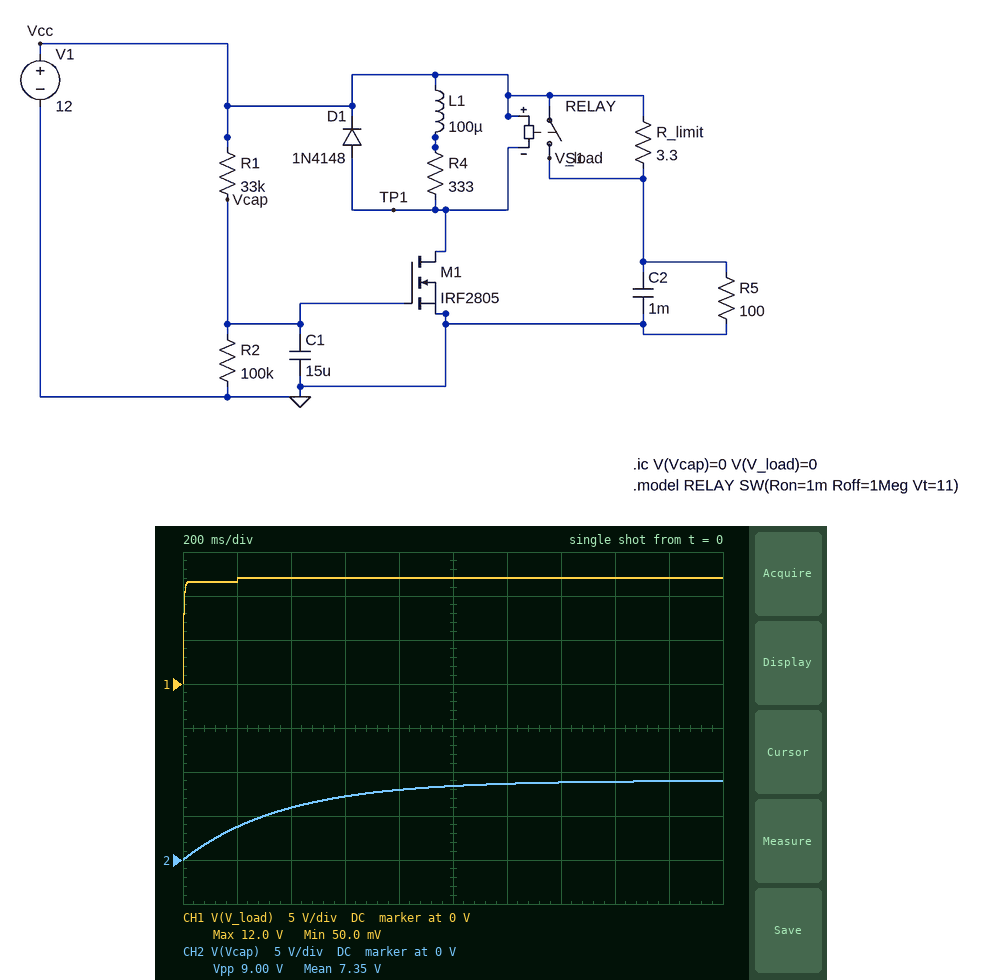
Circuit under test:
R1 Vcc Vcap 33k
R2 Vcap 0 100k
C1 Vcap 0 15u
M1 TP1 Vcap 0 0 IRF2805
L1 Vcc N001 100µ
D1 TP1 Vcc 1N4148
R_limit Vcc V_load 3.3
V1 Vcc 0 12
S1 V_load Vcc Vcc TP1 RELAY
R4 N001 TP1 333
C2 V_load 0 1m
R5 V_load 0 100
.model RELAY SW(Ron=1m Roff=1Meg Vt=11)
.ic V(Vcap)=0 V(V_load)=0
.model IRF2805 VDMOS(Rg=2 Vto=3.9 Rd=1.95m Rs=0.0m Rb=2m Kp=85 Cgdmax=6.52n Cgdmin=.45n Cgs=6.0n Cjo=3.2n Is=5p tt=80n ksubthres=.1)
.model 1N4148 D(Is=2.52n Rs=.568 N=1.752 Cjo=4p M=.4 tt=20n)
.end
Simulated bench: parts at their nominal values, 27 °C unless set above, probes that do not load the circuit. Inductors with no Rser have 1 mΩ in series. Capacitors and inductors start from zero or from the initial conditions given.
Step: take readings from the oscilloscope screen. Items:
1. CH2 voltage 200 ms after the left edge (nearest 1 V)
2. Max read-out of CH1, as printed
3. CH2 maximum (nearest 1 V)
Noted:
4 V
12.0 V
9 V
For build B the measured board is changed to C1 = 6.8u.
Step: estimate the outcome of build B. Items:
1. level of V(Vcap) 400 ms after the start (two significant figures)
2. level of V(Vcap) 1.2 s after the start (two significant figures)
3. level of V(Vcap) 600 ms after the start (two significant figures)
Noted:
8.2 V
9.0 V
8.8 V
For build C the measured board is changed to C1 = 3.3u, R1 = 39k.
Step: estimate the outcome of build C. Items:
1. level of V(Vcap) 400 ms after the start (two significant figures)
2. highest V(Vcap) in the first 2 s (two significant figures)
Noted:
8.5 V
8.6 V
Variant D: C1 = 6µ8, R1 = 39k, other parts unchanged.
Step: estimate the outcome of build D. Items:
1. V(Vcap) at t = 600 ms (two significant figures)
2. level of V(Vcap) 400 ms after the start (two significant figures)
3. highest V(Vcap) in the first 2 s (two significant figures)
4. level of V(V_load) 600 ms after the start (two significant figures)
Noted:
8.3 V
7.6 V
8.6 V
12 V
